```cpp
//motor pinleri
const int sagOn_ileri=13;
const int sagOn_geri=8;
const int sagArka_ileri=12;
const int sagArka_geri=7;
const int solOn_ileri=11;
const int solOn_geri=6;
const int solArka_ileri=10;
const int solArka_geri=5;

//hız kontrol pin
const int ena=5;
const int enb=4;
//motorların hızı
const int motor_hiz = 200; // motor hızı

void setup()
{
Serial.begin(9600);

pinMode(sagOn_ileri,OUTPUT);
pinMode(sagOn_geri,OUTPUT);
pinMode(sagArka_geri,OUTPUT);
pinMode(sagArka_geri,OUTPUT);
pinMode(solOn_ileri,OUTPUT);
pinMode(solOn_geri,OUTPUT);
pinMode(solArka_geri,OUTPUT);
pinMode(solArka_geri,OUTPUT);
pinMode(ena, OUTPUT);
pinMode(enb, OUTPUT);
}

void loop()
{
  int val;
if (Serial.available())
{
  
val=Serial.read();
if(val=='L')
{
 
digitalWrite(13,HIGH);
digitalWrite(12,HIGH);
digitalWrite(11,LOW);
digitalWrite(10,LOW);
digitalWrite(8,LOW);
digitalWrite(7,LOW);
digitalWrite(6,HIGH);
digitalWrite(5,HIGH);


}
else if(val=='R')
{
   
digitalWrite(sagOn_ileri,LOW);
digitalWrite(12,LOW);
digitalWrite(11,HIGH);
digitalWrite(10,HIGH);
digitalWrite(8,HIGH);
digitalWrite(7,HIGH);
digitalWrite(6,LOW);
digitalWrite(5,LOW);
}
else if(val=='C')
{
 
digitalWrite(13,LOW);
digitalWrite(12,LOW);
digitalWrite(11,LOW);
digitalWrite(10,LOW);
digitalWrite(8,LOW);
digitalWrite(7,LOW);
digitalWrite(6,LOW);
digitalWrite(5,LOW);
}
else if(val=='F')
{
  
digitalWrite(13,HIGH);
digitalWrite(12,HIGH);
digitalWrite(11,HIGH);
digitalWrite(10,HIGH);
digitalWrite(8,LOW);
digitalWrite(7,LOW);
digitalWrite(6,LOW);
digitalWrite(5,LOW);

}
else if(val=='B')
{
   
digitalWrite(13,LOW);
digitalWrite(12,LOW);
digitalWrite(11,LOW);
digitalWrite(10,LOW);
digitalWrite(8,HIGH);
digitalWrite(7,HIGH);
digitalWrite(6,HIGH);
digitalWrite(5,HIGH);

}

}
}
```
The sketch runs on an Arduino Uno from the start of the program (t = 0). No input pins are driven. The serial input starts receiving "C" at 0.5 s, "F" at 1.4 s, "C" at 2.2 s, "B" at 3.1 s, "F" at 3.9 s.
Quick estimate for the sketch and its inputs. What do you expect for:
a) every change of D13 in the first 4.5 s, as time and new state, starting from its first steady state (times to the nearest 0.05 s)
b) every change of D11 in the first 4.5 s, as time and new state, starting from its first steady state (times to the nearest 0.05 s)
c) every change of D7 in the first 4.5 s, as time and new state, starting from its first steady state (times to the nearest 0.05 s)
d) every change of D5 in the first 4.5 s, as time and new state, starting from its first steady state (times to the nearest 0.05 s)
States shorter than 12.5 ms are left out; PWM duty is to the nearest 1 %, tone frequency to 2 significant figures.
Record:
0 s low; 1.4 s high; 2.2 s low; 3.9 s high
0 s low; 1.4 s high; 2.2 s low; 3.9 s high
0 s low; 3.1 s high; 3.9 s low
0 s low; 3.1 s high; 3.9 s low
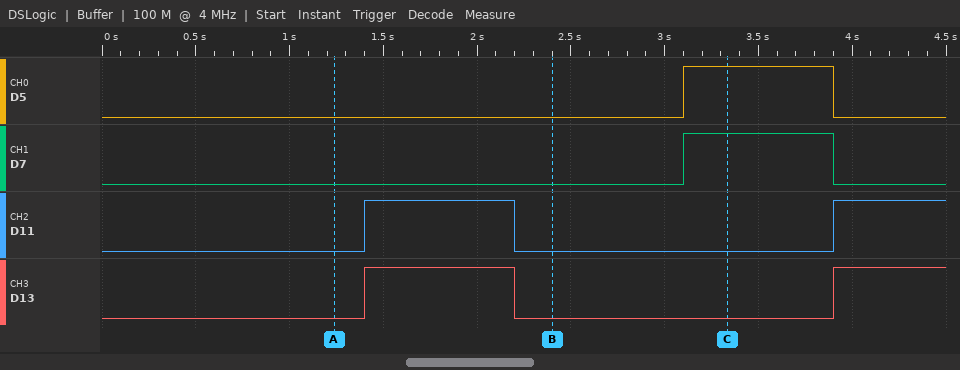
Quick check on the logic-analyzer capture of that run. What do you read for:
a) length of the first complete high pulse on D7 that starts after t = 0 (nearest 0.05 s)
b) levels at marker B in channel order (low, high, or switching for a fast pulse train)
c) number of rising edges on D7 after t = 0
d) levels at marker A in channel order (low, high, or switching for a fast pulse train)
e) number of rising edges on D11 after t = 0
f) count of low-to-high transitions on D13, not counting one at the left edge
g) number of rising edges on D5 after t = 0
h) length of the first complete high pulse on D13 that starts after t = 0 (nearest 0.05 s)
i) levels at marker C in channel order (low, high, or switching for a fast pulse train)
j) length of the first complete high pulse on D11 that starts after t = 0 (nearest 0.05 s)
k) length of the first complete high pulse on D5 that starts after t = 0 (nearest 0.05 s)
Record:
0.80 s
D5 low, D7 low, D11 low, D13 low
1
D5 low, D7 low, D11 low, D13 low
2
2
1
0.80 s
D5 high, D7 high, D11 low, D13 low
0.80 s
0.80 s
